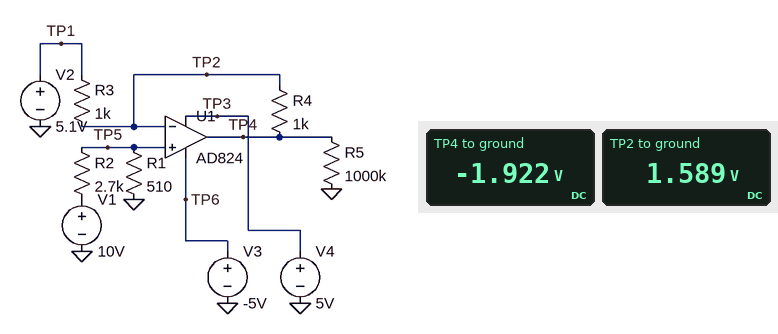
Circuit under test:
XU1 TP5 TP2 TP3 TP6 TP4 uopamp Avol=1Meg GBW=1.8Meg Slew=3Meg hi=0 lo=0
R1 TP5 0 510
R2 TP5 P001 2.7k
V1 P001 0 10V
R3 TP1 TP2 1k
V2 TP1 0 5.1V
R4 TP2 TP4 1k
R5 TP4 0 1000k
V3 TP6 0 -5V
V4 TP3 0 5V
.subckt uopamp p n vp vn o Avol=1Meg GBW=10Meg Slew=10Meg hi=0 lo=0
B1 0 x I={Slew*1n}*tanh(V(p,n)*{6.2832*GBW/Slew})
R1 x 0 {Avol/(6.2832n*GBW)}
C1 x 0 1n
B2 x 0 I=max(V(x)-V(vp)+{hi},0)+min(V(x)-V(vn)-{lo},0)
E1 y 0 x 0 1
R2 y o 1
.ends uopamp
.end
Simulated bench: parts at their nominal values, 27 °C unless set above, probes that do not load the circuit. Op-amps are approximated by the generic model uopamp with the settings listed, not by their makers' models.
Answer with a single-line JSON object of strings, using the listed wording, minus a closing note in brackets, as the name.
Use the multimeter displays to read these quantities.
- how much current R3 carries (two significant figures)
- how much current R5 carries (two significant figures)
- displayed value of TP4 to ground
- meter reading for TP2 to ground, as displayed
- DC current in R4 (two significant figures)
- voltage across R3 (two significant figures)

{"how much current R3 carries": "3.5 mA", "how much current R5 carries": "1.9 µA", "displayed value of TP4 to ground": "-1.922 V", "meter reading for TP2 to ground, as displayed": "1.589 V", "DC current in R4": "3.5 mA", "voltage across R3": "3.5 V"}
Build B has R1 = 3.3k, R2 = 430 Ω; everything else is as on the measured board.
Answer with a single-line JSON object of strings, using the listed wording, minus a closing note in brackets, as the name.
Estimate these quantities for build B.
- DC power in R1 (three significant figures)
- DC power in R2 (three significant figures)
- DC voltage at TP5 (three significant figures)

{"DC power in R1": "23.7 mW", "DC power in R2": "3.09 mW", "DC voltage at TP5": "8.85 V"}
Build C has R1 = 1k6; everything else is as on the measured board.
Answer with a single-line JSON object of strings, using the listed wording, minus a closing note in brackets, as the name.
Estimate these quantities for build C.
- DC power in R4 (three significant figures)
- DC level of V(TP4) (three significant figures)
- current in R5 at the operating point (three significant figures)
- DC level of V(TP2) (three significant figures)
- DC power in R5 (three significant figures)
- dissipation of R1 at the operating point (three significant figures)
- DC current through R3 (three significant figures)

{"DC power in R4": "1.90 mW", "DC level of V(TP4)": "2.34 V", "current in R5 at the operating point": "2.34 µA", "DC level of V(TP2)": "3.72 V", "DC power in R5": "5.48 µW", "dissipation of R1 at the operating point": "8.65 mW", "DC current through R3": "1.38 mA"}
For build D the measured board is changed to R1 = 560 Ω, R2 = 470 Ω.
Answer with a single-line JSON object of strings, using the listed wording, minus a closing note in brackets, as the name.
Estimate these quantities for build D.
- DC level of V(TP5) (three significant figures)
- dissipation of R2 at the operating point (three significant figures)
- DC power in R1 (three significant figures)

{"DC level of V(TP5)": "5.44 V", "dissipation of R2 at the operating point": "44.3 mW", "DC power in R1": "52.8 mW"}
